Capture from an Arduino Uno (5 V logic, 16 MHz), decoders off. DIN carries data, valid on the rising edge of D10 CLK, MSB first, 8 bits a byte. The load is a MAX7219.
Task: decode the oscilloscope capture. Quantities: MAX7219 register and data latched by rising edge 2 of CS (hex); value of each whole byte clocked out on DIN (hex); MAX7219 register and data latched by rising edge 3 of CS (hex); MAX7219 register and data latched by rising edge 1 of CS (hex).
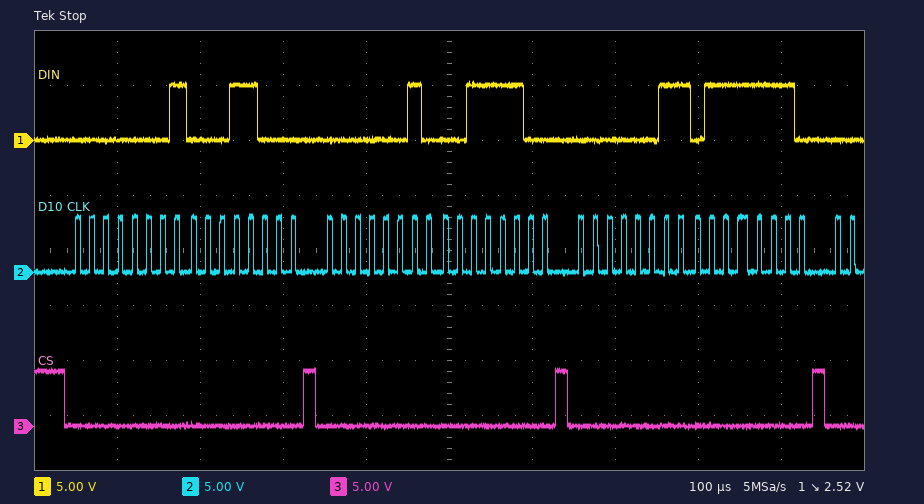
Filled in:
register 0x2, data 0x3C
01 18 02 3C 03 7E
register 0x3, data 0x7E
register 0x1, data 0x18
